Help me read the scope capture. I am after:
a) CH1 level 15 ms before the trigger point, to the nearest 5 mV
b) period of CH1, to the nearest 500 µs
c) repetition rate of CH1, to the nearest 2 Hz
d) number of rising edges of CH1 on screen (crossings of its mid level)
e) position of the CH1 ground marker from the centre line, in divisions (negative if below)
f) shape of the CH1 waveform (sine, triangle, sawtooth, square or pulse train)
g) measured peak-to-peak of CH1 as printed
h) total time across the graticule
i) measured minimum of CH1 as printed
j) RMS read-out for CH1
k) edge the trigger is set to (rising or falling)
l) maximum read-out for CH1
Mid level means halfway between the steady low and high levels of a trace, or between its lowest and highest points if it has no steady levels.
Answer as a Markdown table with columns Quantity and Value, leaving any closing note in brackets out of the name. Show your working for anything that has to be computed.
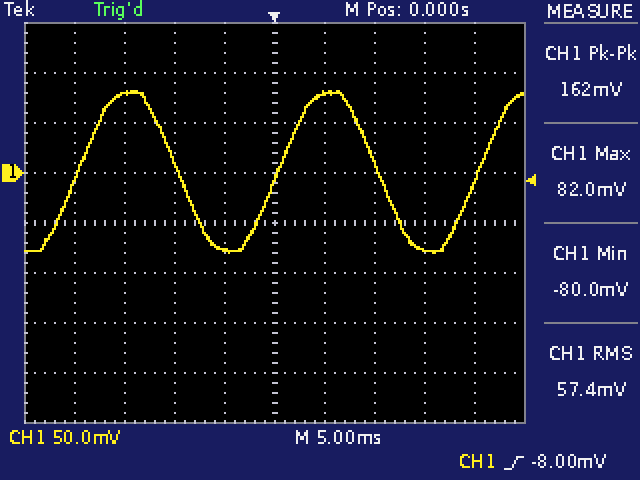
| Quantity | Value |
|---|---|
| CH1 level 15 ms before the trigger point, to the nearest 5 mV | 80 mV |
| period of CH1, to the nearest 500 µs | 20.0 ms |
| repetition rate of CH1, to the nearest 2 Hz | 1 / 20.0 ms ≈ 50 Hz |
| number of rising edges of CH1 on screen | 3 |
| position of the CH1 ground marker from the centre line, in divisions | +1.0 div |
| shape of the CH1 waveform | sine |
| measured peak-to-peak of CH1 as printed | 162 mV |
| total time across the graticule | 50 ms |
| measured minimum of CH1 as printed | -80.0 mV |
| RMS read-out for CH1 | 57.4 mV |
| edge the trigger is set to | rising |
| maximum read-out for CH1 | 82.0 mV |
